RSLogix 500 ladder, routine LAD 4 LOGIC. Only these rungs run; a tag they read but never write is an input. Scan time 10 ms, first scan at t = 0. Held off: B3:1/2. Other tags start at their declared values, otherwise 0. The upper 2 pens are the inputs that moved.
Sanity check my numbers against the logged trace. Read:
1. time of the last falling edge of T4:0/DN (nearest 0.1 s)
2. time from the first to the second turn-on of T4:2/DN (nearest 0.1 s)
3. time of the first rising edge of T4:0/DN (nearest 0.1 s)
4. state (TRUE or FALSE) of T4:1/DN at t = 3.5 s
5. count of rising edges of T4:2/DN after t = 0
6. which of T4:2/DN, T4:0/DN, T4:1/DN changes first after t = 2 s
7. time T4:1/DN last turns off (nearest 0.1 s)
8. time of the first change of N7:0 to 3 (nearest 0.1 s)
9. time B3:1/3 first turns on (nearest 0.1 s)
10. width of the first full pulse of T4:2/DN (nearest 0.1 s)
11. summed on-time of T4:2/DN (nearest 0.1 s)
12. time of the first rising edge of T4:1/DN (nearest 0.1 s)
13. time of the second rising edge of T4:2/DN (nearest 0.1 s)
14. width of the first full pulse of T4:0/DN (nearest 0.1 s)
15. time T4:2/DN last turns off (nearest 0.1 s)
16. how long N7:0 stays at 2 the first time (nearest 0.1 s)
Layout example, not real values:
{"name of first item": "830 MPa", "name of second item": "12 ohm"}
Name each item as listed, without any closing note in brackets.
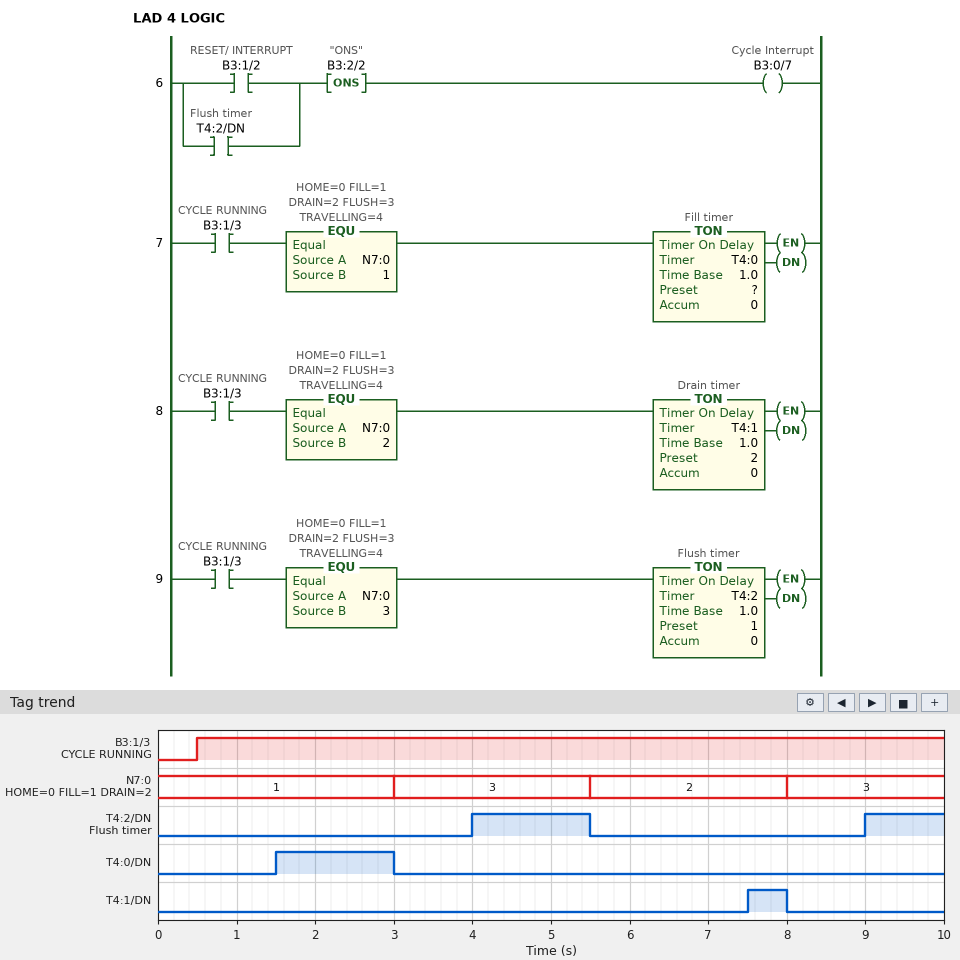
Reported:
{"time of the last falling edge of T4:0/DN": "3.0 s", "time from the first to the second turn-on of T4:2/DN": "5.0 s", "time of the first rising edge of T4:0/DN": "1.5 s", "state (TRUE or FALSE) of T4:1/DN at t = 3.5 s": "FALSE", "count of rising edges of T4:2/DN after t = 0": "2", "which of T4:2/DN, T4:0/DN, T4:1/DN changes first after t = 2 s": "T4:0/DN", "time T4:1/DN last turns off": "8.0 s", "time of the first change of N7:0 to 3": "3.0 s", "time B3:1/3 first turns on": "0.5 s", "width of the first full pulse of T4:2/DN": "1.5 s", "summed on-time of T4:2/DN": "2.5 s", "time of the first rising edge of T4:1/DN": "7.5 s", "time of the second rising edge of T4:2/DN": "9.0 s", "width of the first full pulse of T4:0/DN": "1.5 s", "time T4:2/DN last turns off": "5.5 s", "how long N7:0 stays at 2 the first time": "2.5 s"}
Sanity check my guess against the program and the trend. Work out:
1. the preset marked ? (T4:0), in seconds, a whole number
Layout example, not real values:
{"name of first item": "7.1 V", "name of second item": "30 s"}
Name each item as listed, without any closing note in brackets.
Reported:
{"the preset marked ? (T4:0), in seconds, a whole number": "1 s"}
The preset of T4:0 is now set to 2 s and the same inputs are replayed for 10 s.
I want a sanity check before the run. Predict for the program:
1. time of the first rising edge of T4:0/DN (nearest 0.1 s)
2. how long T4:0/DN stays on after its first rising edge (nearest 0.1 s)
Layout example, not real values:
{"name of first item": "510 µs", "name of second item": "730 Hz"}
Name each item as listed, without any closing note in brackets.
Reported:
{"time of the first rising edge of T4:0/DN": "2.5 s", "how long T4:0/DN stays on after its first rising edge": "0.5 s"}
